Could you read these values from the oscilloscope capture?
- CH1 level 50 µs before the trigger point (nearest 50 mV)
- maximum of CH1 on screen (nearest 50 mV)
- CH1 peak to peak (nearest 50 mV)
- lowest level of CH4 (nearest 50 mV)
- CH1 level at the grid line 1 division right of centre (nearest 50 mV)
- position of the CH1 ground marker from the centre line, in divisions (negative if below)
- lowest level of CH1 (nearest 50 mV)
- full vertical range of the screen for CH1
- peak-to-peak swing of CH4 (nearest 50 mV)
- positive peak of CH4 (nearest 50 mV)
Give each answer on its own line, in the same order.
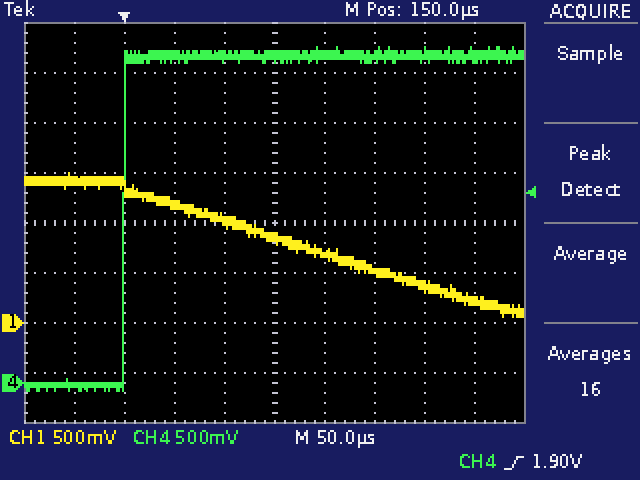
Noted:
1.40 V
1.50 V
1.45 V
-100 mV
700 mV
-2.0 div
50 mV
4 V
3.45 V
3.35 V
